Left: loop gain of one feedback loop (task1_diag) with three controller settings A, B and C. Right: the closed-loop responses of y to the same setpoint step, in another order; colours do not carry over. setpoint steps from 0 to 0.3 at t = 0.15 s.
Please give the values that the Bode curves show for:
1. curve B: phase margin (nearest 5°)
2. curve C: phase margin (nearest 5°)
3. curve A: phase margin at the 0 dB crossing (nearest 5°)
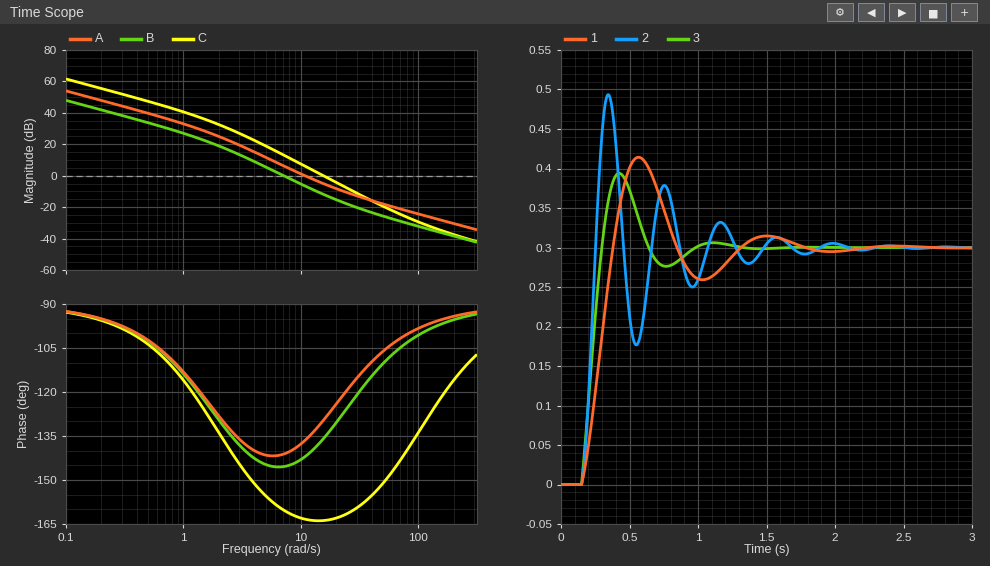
35°
15°
45°
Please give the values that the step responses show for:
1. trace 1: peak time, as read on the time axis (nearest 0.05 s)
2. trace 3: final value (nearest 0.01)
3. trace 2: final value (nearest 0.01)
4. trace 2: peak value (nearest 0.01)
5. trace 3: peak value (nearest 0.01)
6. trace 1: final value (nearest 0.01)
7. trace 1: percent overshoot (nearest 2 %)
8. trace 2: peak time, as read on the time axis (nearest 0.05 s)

0.55 s
0.30
0.30
0.49
0.39
0.30
38 %
0.35 s
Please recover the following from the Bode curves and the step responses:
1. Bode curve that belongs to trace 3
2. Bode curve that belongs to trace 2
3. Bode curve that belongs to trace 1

A
C
B
